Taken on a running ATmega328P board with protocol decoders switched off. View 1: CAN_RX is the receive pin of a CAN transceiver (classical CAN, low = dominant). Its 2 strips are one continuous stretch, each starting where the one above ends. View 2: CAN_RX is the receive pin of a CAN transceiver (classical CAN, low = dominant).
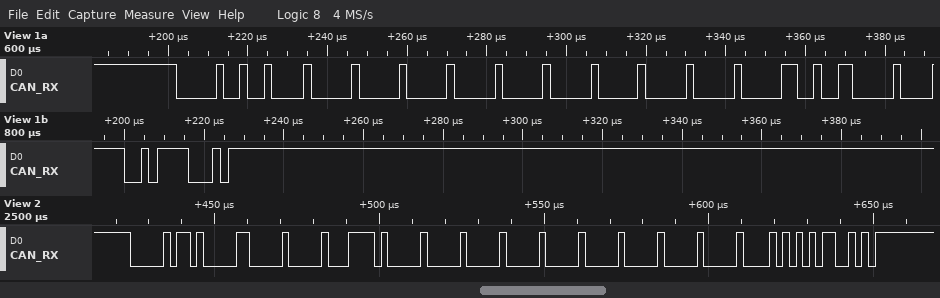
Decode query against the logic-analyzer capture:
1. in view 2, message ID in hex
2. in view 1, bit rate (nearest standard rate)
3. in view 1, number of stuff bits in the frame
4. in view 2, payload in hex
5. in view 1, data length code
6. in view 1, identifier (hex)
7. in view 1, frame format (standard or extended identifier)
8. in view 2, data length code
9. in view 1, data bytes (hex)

0x034
500 kbit/s
12
00 3D 00 00 00 00 00 00
8
0x012
standard
8
00 00 00 00 00 01 26 00
